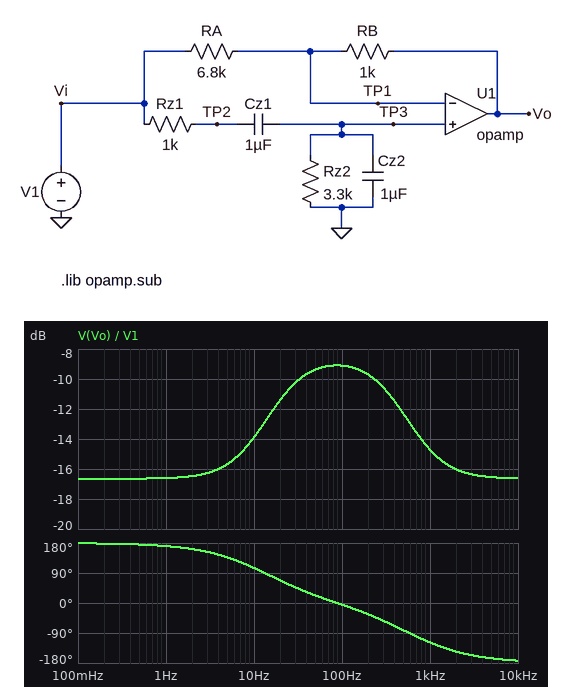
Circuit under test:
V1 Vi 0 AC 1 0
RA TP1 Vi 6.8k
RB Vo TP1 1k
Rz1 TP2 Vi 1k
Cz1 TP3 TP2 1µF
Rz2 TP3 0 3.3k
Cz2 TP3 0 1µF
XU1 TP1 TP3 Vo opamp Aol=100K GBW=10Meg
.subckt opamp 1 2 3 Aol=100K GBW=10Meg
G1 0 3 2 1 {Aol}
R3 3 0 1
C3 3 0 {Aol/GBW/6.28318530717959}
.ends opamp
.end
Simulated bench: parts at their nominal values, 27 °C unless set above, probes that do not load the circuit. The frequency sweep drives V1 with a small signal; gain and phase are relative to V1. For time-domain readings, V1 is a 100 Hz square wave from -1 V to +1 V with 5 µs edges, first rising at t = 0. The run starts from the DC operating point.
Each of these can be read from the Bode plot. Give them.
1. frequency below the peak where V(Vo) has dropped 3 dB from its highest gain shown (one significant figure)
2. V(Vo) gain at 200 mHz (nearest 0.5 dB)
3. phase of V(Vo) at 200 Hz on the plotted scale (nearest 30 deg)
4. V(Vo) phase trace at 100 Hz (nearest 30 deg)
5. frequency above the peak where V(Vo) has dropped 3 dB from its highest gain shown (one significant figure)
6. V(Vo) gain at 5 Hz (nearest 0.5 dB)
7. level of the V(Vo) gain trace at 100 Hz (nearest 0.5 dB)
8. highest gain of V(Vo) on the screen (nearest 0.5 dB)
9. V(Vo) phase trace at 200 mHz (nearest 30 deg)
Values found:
20 Hz
-16.5 dB
-30 deg
0 deg
500 Hz
-15.5 dB
-9.0 dB
-9.0 dB
180 deg
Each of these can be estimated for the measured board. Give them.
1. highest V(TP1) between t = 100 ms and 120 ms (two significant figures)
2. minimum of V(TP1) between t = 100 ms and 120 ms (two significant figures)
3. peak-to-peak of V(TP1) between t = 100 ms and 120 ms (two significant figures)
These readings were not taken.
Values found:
500 mV
-500 mV
990 mV
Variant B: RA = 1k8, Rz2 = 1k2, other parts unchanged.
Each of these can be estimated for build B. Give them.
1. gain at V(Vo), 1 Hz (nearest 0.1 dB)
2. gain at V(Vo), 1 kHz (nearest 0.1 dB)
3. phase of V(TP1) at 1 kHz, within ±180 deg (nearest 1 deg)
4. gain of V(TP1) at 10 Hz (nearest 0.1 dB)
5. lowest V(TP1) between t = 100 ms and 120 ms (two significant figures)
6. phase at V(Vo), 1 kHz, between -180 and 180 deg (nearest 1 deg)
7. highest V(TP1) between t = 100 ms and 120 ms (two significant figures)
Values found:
-5.1 dB
-5.9 dB
-65 deg
-22.6 dB
-480 mV
-156 deg
480 mV
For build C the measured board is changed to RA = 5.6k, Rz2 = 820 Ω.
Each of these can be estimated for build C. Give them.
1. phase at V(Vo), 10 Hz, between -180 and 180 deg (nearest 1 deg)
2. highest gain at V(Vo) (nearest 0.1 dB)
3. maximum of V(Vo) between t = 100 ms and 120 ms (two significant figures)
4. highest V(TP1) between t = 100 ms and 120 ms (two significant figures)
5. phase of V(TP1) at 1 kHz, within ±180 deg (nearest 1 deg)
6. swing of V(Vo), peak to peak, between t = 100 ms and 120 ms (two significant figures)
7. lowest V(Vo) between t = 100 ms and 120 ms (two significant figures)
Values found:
161 deg
-14.5 dB
350 mV
450 mV
-62 deg
700 mV
-350 mV
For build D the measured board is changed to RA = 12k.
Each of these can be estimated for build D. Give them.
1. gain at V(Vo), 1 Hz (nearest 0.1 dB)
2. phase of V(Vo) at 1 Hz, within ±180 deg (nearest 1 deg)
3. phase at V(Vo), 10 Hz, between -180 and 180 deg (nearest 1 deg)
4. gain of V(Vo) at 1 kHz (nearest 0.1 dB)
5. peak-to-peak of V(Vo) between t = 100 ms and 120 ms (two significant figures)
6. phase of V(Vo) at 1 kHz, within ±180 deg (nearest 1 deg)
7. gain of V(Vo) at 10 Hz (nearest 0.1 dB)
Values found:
-21.4 dB
165 deg
88 deg
-16.2 dB
910 mV
-100 deg
-14.7 dB
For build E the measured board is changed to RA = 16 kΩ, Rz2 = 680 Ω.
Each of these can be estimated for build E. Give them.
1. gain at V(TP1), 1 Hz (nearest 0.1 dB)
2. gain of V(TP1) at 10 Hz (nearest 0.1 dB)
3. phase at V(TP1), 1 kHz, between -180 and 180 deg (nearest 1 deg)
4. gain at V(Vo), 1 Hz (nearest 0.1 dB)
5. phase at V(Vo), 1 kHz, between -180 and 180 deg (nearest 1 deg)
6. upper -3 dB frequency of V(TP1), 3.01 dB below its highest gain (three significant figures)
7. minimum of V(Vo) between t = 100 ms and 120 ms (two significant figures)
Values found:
-47.4 dB
-27.5 dB
-60 deg
-24.1 dB
-84 deg
613 Hz
-390 mV
